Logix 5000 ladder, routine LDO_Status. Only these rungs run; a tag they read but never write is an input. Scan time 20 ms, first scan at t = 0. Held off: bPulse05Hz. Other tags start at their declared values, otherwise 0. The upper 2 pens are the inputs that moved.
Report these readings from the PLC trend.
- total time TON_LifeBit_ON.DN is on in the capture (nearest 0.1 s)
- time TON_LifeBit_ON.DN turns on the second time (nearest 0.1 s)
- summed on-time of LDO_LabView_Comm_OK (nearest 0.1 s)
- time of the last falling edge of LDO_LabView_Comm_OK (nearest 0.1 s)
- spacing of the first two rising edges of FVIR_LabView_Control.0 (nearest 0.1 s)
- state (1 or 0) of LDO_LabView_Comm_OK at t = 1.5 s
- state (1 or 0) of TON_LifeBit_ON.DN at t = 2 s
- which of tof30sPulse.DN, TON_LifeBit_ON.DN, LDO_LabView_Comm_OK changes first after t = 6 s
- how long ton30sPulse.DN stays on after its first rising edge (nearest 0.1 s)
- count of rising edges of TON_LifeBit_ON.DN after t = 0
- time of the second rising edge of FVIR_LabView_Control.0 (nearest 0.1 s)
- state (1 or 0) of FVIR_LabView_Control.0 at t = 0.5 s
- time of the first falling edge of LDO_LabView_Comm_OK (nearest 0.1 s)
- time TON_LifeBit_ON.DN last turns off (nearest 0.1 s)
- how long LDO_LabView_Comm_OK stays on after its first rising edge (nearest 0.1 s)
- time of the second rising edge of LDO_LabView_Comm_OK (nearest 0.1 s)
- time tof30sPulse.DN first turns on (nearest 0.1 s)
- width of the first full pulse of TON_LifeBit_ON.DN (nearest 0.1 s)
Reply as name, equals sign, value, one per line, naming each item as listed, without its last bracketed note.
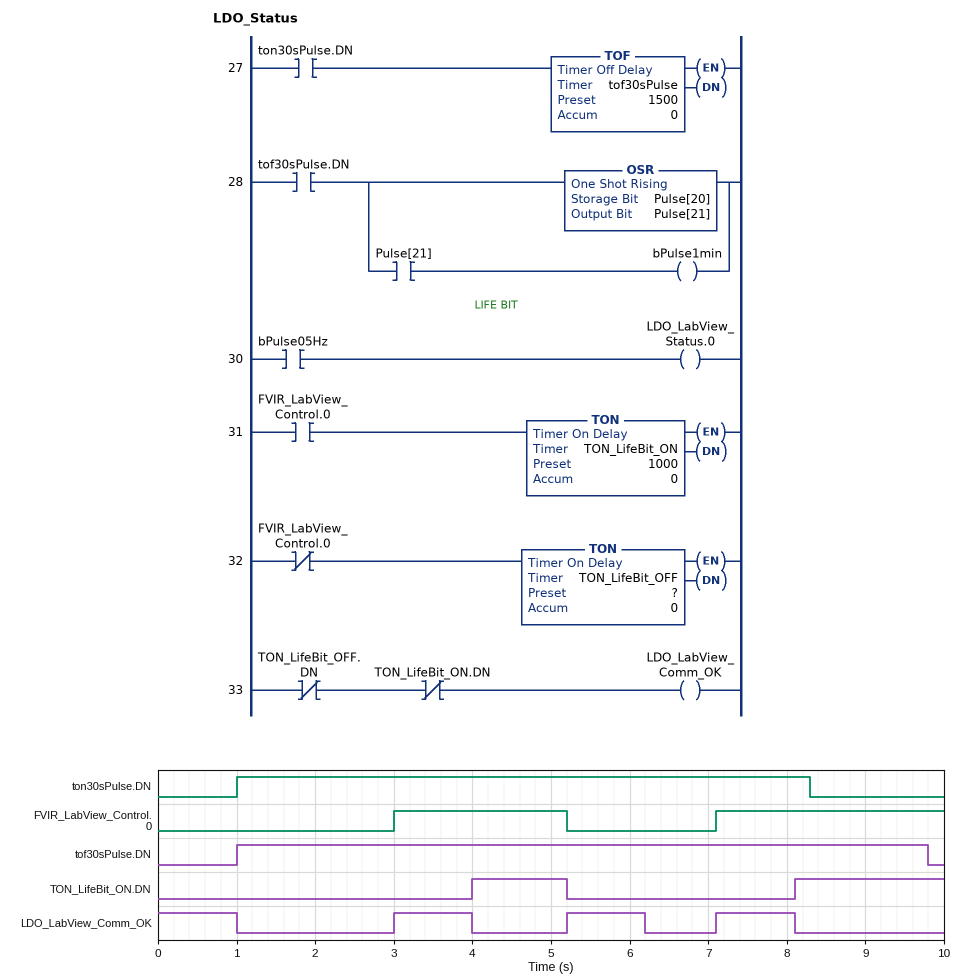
total time TON_LifeBit_ON.DN is on in the capture = 3.1 s
time TON_LifeBit_ON.DN turns on the second time = 8.1 s
summed on-time of LDO_LabView_Comm_OK = 4.0 s
time of the last falling edge of LDO_LabView_Comm_OK = 8.1 s
spacing of the first two rising edges of FVIR_LabView_Control.0 = 4.1 s
state (1 or 0) of LDO_LabView_Comm_OK at t = 1.5 s = 0
state (1 or 0) of TON_LifeBit_ON.DN at t = 2 s = 0
which of tof30sPulse.DN, TON_LifeBit_ON.DN, LDO_LabView_Comm_OK changes first after t = 6 s = LDO_LabView_Comm_OK
how long ton30sPulse.DN stays on after its first rising edge = 7.3 s
count of rising edges of TON_LifeBit_ON.DN after t = 0 = 2
time of the second rising edge of FVIR_LabView_Control.0 = 7.1 s
state (1 or 0) of FVIR_LabView_Control.0 at t = 0.5 s = 0
time of the first falling edge of LDO_LabView_Comm_OK = 1.0 s
time TON_LifeBit_ON.DN last turns off = 5.2 s
how long LDO_LabView_Comm_OK stays on after its first rising edge = 1.0 s
time of the second rising edge of LDO_LabView_Comm_OK = 5.2 s
time tof30sPulse.DN first turns on = 1.0 s
width of the first full pulse of TON_LifeBit_ON.DN = 1.2 s
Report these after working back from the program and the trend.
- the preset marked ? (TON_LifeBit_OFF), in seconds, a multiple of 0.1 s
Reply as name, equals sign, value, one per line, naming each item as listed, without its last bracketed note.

the preset marked ? (TON_LifeBit_OFF), in seconds, a multiple of 0.1 s = 1.0 s
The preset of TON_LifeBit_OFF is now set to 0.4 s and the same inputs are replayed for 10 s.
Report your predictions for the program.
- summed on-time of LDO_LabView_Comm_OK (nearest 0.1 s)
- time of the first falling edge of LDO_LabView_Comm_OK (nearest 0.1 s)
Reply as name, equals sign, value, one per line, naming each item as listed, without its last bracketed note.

summed on-time of LDO_LabView_Comm_OK = 2.8 s
time of the first falling edge of LDO_LabView_Comm_OK = 0.4 s
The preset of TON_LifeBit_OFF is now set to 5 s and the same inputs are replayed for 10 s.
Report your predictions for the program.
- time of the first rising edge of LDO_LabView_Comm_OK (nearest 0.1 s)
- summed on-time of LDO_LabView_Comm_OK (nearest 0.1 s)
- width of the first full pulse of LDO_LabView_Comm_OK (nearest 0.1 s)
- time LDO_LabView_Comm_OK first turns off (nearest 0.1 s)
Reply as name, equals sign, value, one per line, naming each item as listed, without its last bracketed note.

time of the first rising edge of LDO_LabView_Comm_OK = 5.2 s
summed on-time of LDO_LabView_Comm_OK = 6.9 s
width of the first full pulse of LDO_LabView_Comm_OK = 2.9 s
time LDO_LabView_Comm_OK first turns off = 4.0 s
